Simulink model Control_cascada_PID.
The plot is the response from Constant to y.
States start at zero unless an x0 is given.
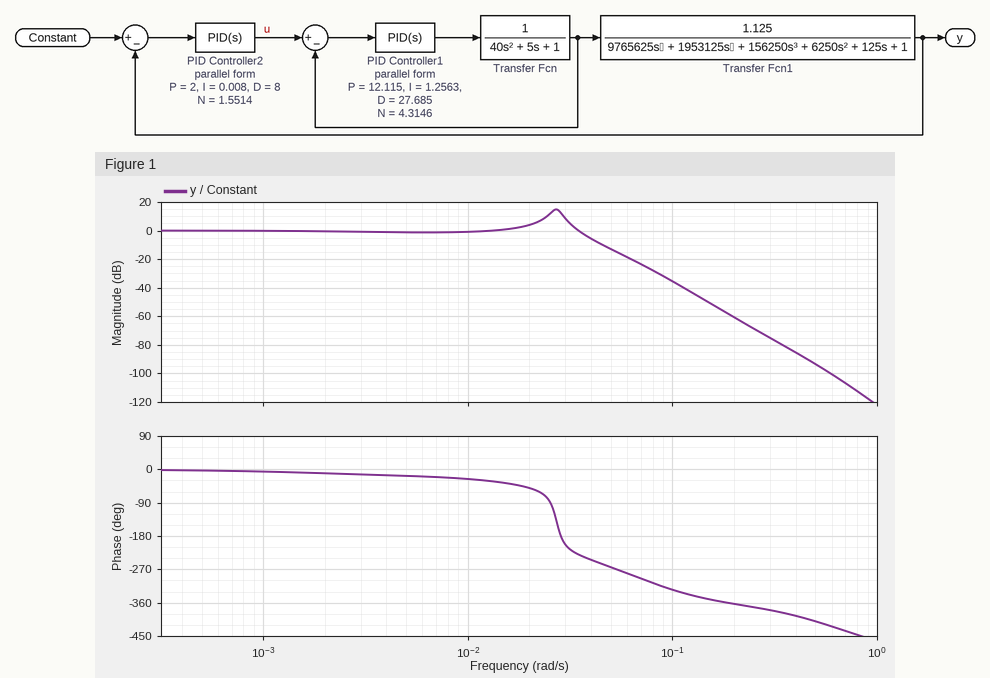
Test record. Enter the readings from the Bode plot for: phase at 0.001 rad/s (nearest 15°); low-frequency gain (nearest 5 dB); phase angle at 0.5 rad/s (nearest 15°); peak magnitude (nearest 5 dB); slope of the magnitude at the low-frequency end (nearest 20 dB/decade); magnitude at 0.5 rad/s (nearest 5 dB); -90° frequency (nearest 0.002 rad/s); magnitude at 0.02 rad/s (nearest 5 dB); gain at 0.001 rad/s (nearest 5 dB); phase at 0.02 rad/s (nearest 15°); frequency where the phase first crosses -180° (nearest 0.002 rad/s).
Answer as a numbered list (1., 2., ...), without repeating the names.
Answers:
1. 0°
2. 0 dB
3. -405°
4. 15 dB
5. 0 dB/decade
6. -95 dB
7. 0.026 rad/s
8. 5 dB
9. 0 dB
10. -45°
11. 0.028 rad/s
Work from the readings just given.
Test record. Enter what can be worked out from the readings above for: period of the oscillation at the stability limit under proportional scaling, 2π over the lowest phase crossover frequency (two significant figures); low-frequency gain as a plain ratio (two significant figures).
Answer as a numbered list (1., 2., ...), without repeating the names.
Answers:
1. 220 s
2. 1.0
